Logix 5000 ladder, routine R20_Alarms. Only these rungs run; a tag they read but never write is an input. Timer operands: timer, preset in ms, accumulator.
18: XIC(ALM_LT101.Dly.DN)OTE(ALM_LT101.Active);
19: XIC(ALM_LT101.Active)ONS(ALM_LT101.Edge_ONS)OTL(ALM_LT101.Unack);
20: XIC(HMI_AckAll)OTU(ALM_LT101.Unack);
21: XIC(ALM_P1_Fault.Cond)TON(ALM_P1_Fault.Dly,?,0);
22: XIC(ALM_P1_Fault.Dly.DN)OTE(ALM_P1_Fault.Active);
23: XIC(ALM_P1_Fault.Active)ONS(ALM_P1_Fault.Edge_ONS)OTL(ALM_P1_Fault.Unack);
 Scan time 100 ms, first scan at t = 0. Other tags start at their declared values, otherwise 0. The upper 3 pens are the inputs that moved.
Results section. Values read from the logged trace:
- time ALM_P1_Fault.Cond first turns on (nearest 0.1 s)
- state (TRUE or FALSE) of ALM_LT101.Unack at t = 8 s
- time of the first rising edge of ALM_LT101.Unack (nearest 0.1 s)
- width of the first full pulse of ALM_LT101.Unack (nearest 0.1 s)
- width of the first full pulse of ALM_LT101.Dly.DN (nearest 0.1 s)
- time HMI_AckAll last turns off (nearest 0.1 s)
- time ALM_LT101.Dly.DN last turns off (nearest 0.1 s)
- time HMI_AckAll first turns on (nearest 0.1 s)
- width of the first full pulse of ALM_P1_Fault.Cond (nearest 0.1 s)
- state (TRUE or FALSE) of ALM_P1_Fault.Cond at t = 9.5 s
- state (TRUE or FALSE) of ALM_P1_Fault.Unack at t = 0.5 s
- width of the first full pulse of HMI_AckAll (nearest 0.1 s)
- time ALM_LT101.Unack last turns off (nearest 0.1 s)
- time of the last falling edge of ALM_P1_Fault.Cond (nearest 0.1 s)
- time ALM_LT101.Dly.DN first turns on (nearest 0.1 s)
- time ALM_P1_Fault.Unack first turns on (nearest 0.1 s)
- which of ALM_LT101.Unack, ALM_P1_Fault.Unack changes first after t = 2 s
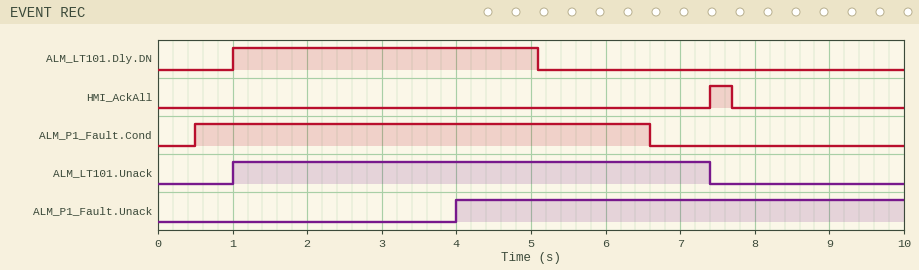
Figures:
0.5 s
FALSE
1.0 s
6.4 s
4.1 s
7.7 s
5.1 s
7.4 s
6.1 s
FALSE
FALSE
0.3 s
7.4 s
6.6 s
1.0 s
4.0 s
ALM_P1_Fault.Unack
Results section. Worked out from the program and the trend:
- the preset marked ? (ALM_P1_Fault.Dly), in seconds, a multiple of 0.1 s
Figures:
3.5 s
